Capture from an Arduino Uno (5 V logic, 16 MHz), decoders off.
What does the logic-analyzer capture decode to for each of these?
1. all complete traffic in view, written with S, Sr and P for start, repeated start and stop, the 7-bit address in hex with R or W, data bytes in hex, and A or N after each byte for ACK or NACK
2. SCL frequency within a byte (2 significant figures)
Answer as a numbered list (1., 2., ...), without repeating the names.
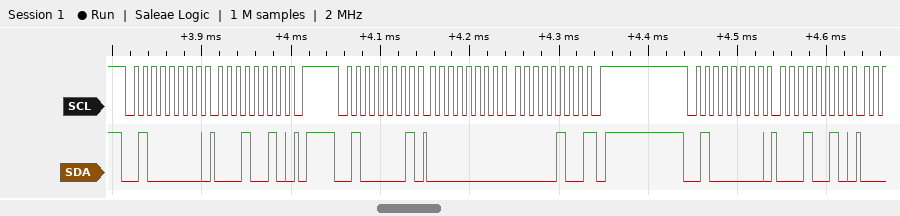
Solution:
1. S 20W A 12 A P S 20R A 00 A 04 N P S 20W A 12 A
2. 100 kHz
